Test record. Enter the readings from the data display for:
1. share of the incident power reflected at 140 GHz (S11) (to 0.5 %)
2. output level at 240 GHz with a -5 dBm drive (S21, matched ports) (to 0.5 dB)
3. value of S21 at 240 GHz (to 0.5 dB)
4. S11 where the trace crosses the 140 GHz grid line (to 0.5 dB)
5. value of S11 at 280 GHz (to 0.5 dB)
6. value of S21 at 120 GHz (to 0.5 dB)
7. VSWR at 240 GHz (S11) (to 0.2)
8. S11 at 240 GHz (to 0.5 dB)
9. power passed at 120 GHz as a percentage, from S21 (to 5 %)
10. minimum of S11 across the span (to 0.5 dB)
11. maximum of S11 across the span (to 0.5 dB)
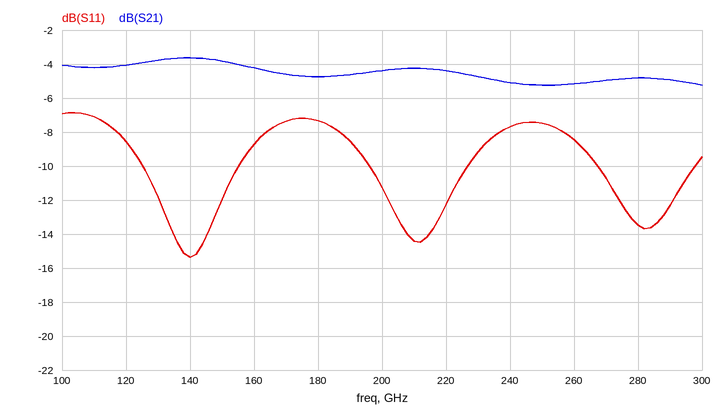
3.0 %
-10.0 dBm
-5.0 dB
-15.5 dB
-13.5 dB
-4.0 dB
2.4
-7.5 dB
40 %
-15.5 dB
-7.0 dB
